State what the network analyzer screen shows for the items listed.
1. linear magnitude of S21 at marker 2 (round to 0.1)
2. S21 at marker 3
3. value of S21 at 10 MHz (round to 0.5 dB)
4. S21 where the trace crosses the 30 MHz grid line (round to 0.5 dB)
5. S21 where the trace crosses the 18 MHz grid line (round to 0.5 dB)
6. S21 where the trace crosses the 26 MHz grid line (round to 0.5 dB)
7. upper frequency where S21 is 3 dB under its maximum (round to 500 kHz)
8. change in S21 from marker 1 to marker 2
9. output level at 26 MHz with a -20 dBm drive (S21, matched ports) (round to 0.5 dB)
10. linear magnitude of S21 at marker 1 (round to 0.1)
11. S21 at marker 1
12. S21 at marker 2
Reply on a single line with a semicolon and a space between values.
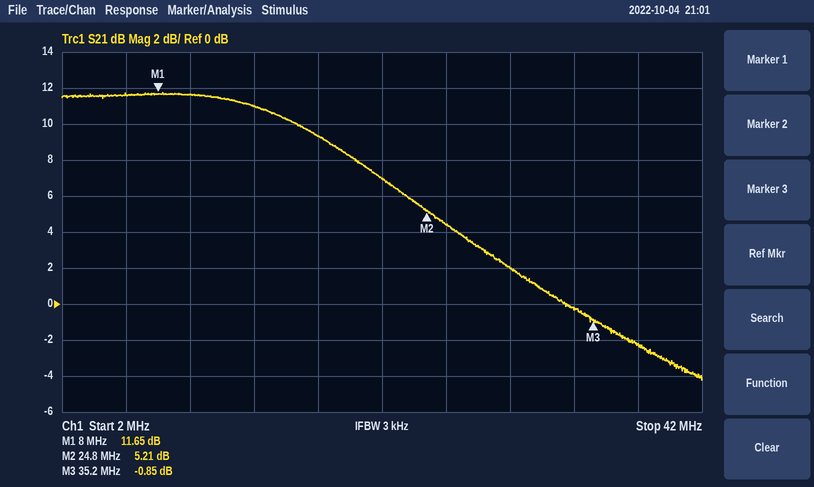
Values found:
1.8; -0.85 dB; 11.5 dB; 2.0 dB; 9.5 dB; 4.5 dB; 19.0 MHz; -6.44 dB; -15.5 dBm; 3.8; 11.65 dB; 5.21 dB
